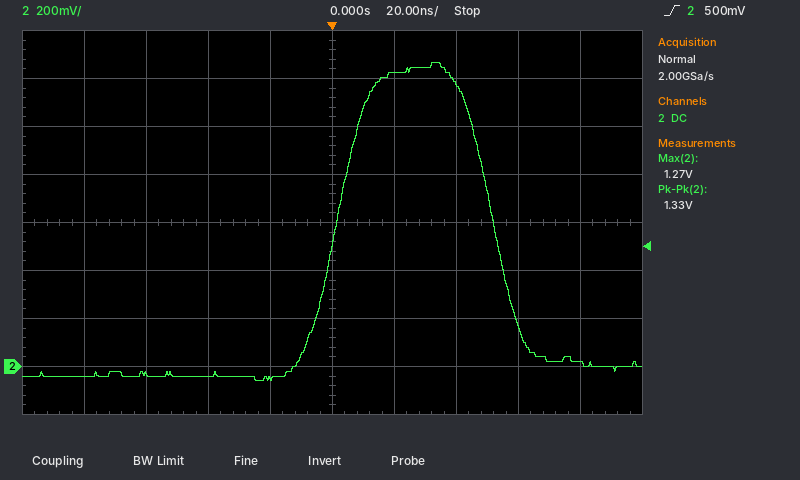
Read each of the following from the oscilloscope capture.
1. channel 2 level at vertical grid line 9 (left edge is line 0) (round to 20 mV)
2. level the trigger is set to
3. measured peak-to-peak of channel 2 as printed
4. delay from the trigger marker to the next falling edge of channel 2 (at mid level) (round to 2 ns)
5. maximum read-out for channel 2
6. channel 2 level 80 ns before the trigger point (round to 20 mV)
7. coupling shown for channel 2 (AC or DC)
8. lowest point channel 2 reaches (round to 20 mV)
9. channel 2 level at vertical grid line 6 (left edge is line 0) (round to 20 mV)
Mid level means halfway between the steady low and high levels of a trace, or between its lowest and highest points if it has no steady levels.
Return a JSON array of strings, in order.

["20 mV", "500 mV", "1.33 V", "52 ns", "1.27 V", "-40 mV", "DC", "-60 mV", "1.22 V"]
